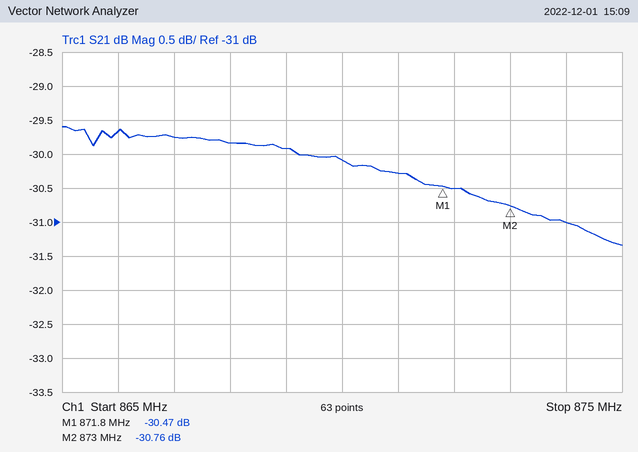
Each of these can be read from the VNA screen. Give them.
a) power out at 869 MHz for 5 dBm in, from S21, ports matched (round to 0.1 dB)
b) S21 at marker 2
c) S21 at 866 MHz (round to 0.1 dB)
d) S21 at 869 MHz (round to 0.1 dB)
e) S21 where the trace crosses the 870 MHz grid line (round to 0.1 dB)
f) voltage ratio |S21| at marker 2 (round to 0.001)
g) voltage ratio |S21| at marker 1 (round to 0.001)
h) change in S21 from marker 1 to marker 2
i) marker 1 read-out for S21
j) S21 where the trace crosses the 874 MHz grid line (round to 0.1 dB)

-24.9 dBm
-30.76 dB
-29.7 dB
-29.9 dB
-30.1 dB
0.029
0.030
-0.29 dB
-30.47 dB
-31.0 dB
